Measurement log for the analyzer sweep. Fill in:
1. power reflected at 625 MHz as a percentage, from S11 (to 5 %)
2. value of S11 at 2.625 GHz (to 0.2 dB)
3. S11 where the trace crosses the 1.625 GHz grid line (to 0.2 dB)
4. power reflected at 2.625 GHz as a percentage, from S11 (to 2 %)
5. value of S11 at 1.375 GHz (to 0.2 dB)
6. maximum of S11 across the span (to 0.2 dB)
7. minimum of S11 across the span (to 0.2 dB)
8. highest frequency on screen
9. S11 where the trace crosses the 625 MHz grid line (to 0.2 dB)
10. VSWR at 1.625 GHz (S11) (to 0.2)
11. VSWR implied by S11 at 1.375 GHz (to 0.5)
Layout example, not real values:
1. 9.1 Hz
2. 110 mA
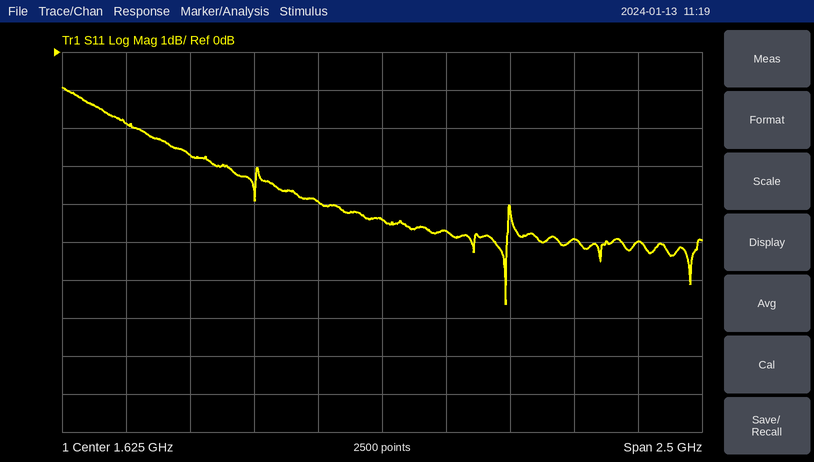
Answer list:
1. 65 %
2. -5.0 dB
3. -4.4 dB
4. 32 %
5. -4.0 dB
6. -1.0 dB
7. -6.6 dB
8. 2.875 GHz
9. -1.8 dB
10. 4.0
11. 4.5
